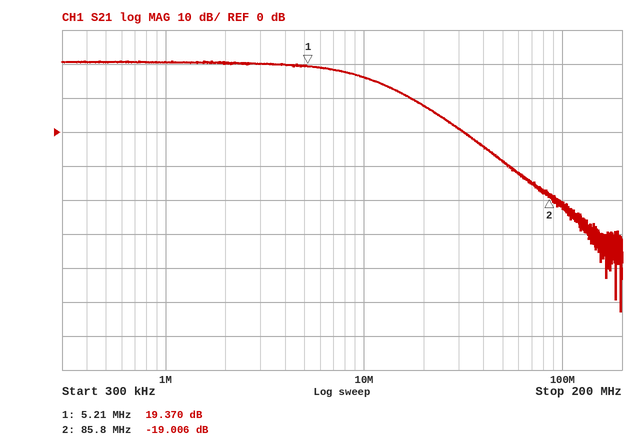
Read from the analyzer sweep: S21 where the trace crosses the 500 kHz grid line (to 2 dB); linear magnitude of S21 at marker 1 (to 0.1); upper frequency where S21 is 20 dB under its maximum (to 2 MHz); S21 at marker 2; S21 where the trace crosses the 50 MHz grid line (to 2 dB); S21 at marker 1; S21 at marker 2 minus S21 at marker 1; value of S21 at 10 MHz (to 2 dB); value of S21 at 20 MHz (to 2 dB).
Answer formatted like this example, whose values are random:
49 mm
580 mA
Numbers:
20 dB
9.3
30 MHz
-19.006 dB
-8 dB
19.370 dB
-38.376 dB
16 dB
8 dB
